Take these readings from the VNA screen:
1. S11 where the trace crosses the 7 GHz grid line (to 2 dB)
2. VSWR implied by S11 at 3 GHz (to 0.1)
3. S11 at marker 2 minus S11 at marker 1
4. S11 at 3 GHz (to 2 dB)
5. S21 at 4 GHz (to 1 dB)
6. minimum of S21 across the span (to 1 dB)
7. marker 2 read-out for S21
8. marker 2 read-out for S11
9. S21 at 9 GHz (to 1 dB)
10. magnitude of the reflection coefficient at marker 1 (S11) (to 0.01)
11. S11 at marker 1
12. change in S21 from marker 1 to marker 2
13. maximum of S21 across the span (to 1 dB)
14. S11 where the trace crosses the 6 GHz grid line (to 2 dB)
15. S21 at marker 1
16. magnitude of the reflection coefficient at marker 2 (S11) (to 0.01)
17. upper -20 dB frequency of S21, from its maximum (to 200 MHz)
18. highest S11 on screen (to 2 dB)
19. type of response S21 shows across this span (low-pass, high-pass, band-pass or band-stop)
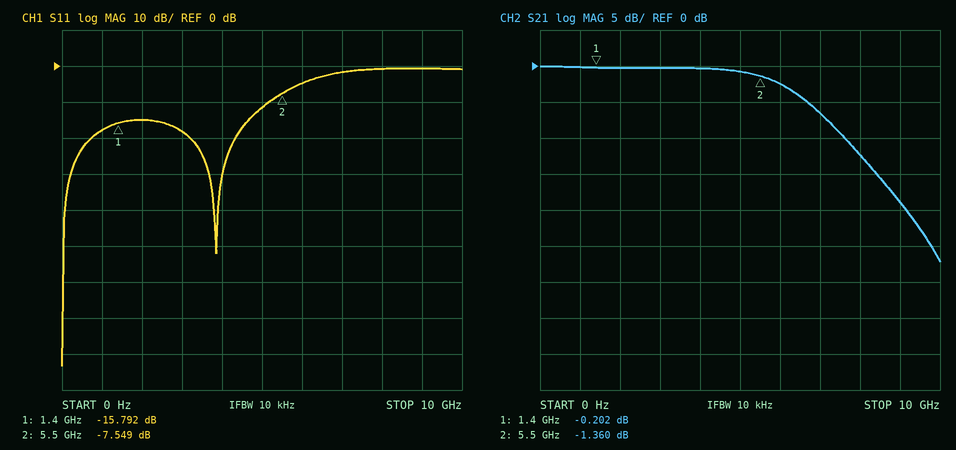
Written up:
-2 dB
1.3
8.243 dB
-18 dB
0 dB
-27 dB
-1.360 dB
-7.549 dB
-19 dB
0.16
-15.792 dB
-1.158 dB
0 dB
-4 dB
-0.202 dB
0.42
9.2 GHz
0 dB
low-pass
